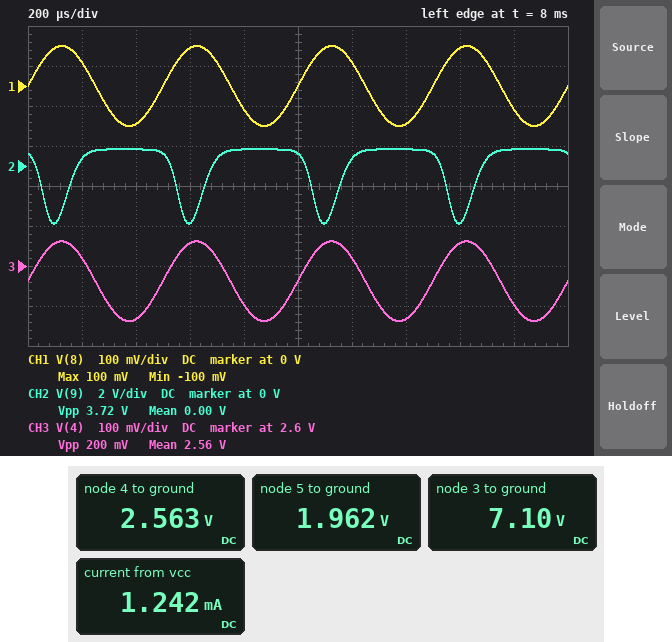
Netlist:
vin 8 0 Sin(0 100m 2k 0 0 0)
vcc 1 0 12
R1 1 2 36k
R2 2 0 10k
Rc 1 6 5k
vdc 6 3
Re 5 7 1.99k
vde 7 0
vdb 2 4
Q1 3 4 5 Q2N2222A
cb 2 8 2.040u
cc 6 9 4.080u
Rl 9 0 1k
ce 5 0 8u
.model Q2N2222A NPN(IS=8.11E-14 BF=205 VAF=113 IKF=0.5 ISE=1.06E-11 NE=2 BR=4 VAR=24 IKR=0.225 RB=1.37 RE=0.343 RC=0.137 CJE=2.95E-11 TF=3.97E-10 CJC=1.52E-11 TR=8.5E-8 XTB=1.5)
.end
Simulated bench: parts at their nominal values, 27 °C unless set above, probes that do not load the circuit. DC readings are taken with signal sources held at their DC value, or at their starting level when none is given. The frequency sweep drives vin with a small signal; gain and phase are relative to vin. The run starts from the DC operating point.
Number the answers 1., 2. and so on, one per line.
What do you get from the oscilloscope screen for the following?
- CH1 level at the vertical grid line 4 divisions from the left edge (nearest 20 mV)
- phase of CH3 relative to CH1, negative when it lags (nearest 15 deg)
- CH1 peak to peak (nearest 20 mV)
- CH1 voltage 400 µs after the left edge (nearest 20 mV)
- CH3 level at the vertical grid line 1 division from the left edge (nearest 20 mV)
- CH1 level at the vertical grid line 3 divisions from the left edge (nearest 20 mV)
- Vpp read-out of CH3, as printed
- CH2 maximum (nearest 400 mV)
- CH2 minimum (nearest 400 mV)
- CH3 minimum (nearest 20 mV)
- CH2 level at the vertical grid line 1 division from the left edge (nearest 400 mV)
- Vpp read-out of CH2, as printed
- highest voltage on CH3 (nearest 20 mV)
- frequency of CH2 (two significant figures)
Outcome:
1. -60 mV
2. 0 deg
3. 200 mV
4. -100 mV
5. 2.62 V
6. 100 mV
7. 200 mV
8. 800 mV
9. -2.8 V
10. 2.46 V
11. 400 mV
12. 3.72 V
13. 2.66 V
14. 2.0 kHz
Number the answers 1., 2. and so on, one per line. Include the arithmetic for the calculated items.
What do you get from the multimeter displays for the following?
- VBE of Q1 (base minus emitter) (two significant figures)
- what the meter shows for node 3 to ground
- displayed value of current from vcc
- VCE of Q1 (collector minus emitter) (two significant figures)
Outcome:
1. 2.563 V - 1.962 V = 600 mV
2. 7.10 V
3. 1.242 mA
4. 7.1 V - 1.962 V = 5.1 V
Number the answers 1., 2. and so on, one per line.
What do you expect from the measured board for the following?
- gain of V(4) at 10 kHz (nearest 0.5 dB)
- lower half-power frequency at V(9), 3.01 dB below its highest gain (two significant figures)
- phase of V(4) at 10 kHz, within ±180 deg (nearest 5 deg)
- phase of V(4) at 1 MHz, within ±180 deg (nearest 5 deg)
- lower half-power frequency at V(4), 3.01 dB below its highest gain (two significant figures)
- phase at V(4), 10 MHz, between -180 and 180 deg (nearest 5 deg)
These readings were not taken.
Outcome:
1. 0 dB
2. 770 Hz
3. 0 deg
4. 0 deg
5. 10 Hz
6. 0 deg
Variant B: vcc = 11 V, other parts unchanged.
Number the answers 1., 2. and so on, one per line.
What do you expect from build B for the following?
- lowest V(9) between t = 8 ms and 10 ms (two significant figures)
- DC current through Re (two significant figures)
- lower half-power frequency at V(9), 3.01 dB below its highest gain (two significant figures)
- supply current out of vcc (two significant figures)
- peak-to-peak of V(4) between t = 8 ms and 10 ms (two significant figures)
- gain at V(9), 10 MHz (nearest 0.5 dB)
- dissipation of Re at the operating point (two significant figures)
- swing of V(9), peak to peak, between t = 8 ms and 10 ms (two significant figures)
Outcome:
1. -2.6 V
2. 880 µA
3. 690 Hz
4. 1.1 mA
5. 200 mV
6. 28.0 dB
7. 1.5 mW
8. 3.4 V
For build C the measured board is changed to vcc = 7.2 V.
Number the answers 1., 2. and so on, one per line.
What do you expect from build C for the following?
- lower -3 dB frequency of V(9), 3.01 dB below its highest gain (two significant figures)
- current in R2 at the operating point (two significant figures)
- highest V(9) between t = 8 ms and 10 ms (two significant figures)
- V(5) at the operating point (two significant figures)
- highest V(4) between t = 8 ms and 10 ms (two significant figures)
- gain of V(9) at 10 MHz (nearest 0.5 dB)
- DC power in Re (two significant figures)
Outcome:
1. 380 Hz
2. 150 µA
3. 420 mV
4. 960 mV
5. 1.6 V
6. 23.0 dB
7. 460 µW
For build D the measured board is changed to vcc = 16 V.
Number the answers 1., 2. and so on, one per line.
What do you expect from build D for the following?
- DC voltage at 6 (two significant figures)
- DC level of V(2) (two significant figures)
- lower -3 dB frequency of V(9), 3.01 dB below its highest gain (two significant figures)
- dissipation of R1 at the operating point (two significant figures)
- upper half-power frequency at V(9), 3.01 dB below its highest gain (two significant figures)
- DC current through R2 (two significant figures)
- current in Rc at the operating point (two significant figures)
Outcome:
1. 9.0 V
2. 3.4 V
3. 1.1 kHz
4. 4.4 mW
5. 24 MHz
6. 340 µA
7. 1.4 mA
